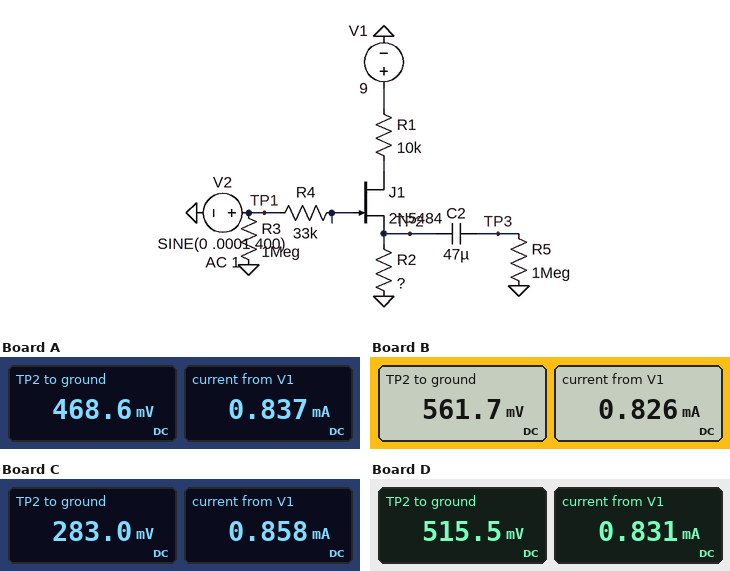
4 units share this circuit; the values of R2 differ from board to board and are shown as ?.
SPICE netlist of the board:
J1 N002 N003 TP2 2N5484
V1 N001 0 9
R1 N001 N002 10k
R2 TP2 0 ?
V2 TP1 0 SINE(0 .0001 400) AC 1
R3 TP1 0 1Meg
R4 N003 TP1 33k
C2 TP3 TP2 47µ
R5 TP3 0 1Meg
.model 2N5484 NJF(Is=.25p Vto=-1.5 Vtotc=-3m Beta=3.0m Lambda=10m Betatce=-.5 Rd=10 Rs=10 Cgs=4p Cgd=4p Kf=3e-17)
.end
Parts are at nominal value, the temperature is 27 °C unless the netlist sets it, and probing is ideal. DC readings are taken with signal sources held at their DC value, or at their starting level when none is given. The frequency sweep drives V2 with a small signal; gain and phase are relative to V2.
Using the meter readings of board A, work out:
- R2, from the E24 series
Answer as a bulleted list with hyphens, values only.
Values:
- 560 Ω
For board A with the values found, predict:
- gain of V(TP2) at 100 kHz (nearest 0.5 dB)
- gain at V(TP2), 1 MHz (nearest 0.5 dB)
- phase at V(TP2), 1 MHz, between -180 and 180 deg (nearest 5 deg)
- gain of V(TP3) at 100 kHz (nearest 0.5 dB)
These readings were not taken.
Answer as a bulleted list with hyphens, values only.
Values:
- -41.0 dB
- -37.0 dB
- 15 deg
- -41.0 dB
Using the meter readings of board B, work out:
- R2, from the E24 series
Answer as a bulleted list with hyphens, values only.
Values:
- 680 Ω
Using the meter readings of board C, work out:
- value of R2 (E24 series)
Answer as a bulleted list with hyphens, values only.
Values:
- 330 Ω
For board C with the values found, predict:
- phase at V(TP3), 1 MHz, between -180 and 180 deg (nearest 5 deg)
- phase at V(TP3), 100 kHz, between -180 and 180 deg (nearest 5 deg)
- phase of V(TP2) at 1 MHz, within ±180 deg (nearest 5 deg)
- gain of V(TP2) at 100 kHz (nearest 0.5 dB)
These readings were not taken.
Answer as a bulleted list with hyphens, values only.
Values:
- 20 deg
- 15 deg
- 20 deg
- -48.5 dB
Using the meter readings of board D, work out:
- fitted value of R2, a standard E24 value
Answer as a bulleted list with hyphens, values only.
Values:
- 620 Ω
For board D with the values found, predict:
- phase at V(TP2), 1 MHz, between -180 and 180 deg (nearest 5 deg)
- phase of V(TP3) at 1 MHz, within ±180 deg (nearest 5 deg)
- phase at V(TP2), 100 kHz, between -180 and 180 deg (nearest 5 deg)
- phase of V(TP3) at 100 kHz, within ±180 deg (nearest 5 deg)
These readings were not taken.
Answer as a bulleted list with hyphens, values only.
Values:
- 10 deg
- 10 deg
- 5 deg
- 5 deg
